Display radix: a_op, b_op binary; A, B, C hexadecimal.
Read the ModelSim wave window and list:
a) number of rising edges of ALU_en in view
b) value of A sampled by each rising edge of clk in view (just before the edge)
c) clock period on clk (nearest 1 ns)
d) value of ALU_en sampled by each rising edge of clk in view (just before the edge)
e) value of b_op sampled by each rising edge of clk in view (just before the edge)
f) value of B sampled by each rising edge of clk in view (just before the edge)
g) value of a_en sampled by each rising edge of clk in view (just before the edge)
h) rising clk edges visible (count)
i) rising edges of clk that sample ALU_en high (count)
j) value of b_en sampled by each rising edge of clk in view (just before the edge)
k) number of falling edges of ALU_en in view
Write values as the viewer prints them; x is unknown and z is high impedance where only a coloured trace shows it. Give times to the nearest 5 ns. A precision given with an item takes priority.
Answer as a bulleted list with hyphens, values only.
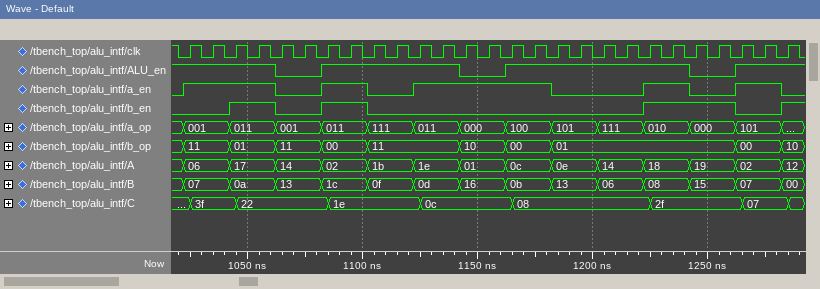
- 3
- 06, 06, 17, 17, 14, 14, 02, 02, 1b, 1b, 1e, 1e, 01, 01, 0c, 0c, 0e, 0e, 14, 14, 18, 18, 19, 19, 02, 02, 12
- 10 ns
- 1 1 1 1 0 0 1 1 1 1 1 1 0 0 1 1 1 1 1 1 1 1 0 0 1 1 1
- 11, 11, 01, 01, 11, 11, 00, 00, 11, 11, 11, 11, 10, 10, 00, 00, 01, 01, 01, 01, 01, 01, 01, 01, 00, 00, 10
- 07, 07, 0a, 0a, 13, 13, 1c, 1c, 0f, 0f, 0d, 0d, 16, 16, 0b, 0b, 13, 13, 06, 06, 08, 08, 15, 15, 07, 07, 00
- 1 1 1 1 0 0 1 1 0 0 1 1 1 1 1 1 0 0 0 0 1 1 0 0 1 1 0
- 27
- 21
- 0 0 1 1 0 0 1 1 0 0 0 0 0 0 0 0 0 0 0 0 1 1 1 1 0 0 1
- 3
